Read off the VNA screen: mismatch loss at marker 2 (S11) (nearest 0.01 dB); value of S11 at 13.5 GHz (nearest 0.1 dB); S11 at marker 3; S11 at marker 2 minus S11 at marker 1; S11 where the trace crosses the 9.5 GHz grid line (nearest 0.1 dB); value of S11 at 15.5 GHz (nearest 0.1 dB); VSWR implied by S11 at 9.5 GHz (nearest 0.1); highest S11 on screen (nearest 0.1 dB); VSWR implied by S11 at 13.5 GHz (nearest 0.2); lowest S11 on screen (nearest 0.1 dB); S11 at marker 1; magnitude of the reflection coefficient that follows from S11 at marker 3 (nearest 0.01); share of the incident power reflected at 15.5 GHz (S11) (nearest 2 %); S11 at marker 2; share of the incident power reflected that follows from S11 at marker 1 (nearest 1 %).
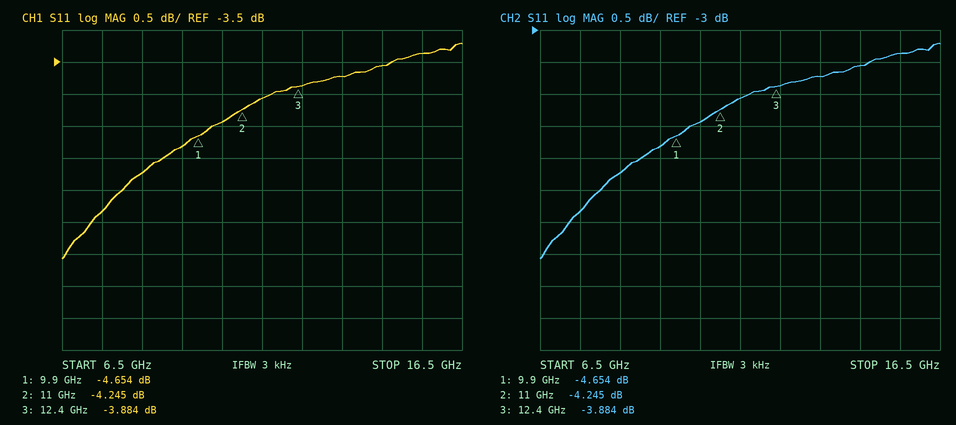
2.05 dB
-3.7 dB
-3.884 dB
0.409 dB
-4.8 dB
-3.4 dB
3.7
-3.2 dB
4.8
-6.6 dB
-4.654 dB
0.64
46 %
-4.245 dB
34 %
